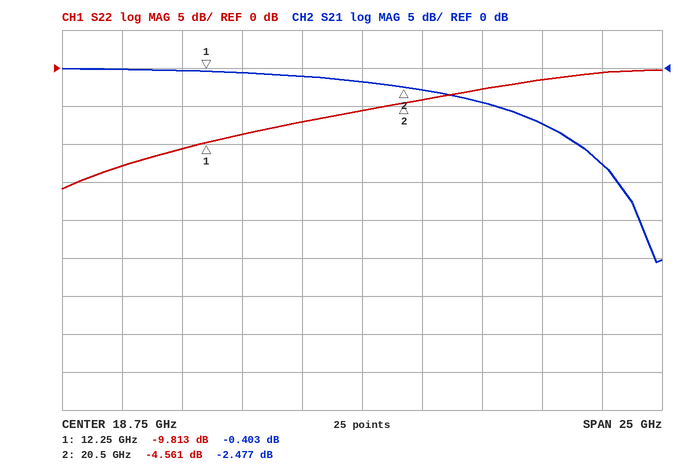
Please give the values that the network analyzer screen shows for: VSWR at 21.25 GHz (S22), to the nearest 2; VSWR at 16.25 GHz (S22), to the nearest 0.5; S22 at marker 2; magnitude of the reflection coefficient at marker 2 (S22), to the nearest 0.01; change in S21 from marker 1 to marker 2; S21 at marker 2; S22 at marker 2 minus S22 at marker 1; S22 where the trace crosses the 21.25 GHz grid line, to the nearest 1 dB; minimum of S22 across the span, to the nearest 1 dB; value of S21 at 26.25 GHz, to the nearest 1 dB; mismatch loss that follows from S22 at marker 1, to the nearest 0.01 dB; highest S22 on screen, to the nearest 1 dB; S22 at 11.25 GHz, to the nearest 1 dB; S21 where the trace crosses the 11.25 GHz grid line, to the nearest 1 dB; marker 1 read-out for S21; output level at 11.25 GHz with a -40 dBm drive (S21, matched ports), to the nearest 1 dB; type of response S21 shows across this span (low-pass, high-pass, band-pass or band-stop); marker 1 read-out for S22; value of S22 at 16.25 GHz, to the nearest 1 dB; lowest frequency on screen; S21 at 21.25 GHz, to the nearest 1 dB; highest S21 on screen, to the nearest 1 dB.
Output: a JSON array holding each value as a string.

["4", "2.5", "-4.561 dB", "0.59", "-2.074 dB", "-2.477 dB", "5.252 dB", "-4 dB", "-16 dB", "-7 dB", "0.48 dB", "0 dB", "-11 dB", "0 dB", "-0.403 dB", "-40 dBm", "low-pass", "-9.813 dB", "-7 dB", "6.25 GHz", "-3 dB", "0 dB"]
